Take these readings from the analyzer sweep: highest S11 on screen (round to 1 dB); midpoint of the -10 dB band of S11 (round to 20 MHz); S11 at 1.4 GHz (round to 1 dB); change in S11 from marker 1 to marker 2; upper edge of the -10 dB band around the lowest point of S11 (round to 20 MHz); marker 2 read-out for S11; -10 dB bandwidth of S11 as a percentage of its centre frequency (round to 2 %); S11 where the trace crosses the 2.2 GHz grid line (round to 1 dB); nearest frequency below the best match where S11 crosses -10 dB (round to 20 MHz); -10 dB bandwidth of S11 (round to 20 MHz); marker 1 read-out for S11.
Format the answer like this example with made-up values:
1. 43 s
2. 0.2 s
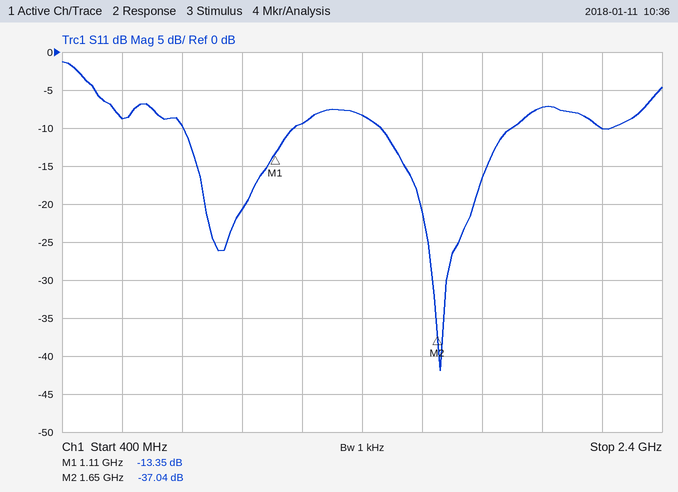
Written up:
1. -1 dB
2. 1.68 GHz
3. -8 dB
4. -23.69 dB
5. 1.90 GHz
6. -37.04 dB
7. 26 %
8. -10 dB
9. 1.46 GHz
10. 440 MHz
11. -13.35 dB
